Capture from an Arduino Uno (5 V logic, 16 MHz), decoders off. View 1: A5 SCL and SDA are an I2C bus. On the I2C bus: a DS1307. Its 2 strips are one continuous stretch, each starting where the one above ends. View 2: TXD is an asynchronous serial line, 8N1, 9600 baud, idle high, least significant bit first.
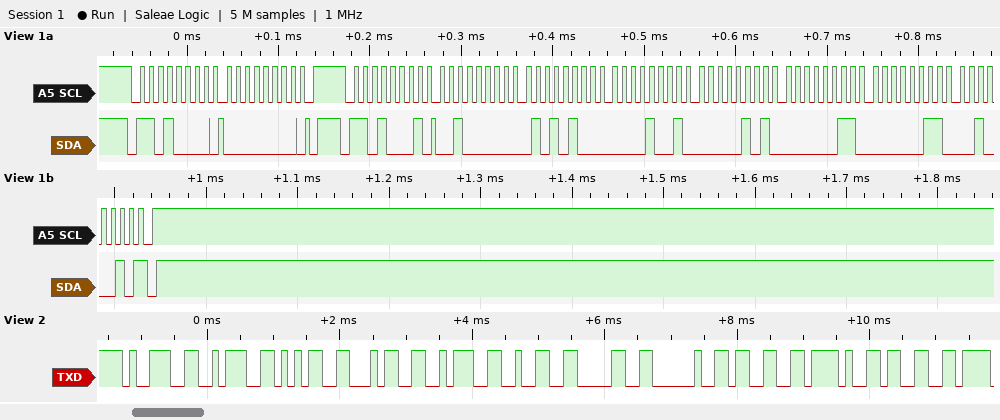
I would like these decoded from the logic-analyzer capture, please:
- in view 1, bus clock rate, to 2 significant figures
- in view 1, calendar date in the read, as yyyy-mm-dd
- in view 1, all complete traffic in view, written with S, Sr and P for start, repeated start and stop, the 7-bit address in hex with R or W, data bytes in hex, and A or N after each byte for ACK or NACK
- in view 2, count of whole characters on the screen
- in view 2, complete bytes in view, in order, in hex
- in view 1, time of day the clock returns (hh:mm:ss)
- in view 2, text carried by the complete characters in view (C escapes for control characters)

100 kHz
2022-03-03
S 68W A 00 A P S 68R A 20 A 54 A 09 A 05 A 03 A 03 A 22 N P
11
39 3A 35 34 3A 32 30 20 33 2F 33
09:54:20
"9:54:20 3/3"
